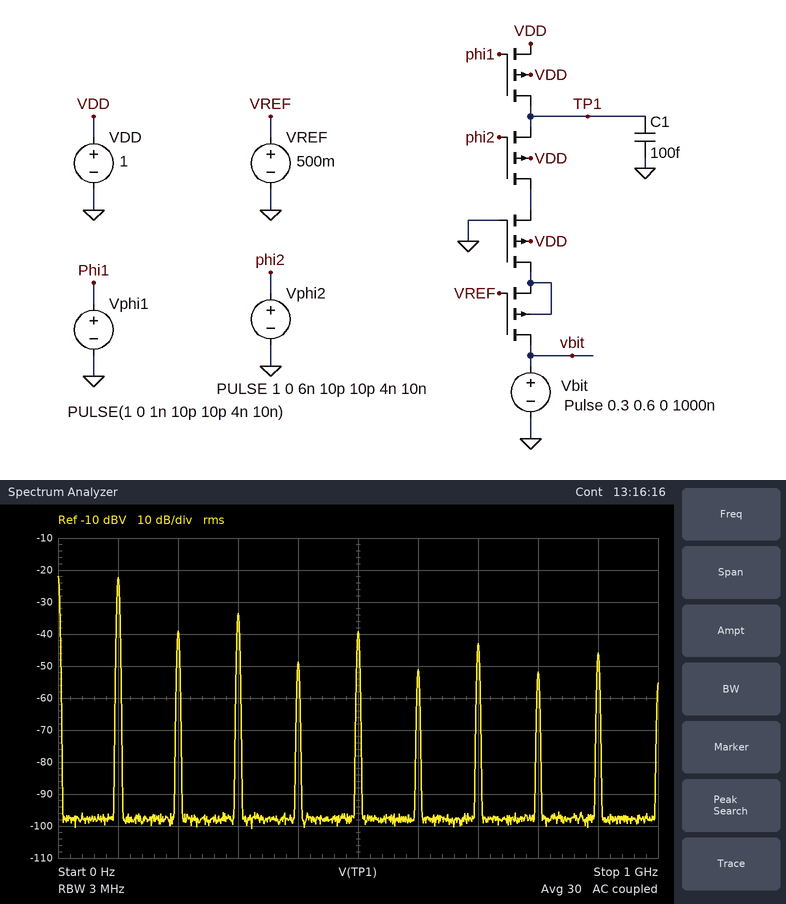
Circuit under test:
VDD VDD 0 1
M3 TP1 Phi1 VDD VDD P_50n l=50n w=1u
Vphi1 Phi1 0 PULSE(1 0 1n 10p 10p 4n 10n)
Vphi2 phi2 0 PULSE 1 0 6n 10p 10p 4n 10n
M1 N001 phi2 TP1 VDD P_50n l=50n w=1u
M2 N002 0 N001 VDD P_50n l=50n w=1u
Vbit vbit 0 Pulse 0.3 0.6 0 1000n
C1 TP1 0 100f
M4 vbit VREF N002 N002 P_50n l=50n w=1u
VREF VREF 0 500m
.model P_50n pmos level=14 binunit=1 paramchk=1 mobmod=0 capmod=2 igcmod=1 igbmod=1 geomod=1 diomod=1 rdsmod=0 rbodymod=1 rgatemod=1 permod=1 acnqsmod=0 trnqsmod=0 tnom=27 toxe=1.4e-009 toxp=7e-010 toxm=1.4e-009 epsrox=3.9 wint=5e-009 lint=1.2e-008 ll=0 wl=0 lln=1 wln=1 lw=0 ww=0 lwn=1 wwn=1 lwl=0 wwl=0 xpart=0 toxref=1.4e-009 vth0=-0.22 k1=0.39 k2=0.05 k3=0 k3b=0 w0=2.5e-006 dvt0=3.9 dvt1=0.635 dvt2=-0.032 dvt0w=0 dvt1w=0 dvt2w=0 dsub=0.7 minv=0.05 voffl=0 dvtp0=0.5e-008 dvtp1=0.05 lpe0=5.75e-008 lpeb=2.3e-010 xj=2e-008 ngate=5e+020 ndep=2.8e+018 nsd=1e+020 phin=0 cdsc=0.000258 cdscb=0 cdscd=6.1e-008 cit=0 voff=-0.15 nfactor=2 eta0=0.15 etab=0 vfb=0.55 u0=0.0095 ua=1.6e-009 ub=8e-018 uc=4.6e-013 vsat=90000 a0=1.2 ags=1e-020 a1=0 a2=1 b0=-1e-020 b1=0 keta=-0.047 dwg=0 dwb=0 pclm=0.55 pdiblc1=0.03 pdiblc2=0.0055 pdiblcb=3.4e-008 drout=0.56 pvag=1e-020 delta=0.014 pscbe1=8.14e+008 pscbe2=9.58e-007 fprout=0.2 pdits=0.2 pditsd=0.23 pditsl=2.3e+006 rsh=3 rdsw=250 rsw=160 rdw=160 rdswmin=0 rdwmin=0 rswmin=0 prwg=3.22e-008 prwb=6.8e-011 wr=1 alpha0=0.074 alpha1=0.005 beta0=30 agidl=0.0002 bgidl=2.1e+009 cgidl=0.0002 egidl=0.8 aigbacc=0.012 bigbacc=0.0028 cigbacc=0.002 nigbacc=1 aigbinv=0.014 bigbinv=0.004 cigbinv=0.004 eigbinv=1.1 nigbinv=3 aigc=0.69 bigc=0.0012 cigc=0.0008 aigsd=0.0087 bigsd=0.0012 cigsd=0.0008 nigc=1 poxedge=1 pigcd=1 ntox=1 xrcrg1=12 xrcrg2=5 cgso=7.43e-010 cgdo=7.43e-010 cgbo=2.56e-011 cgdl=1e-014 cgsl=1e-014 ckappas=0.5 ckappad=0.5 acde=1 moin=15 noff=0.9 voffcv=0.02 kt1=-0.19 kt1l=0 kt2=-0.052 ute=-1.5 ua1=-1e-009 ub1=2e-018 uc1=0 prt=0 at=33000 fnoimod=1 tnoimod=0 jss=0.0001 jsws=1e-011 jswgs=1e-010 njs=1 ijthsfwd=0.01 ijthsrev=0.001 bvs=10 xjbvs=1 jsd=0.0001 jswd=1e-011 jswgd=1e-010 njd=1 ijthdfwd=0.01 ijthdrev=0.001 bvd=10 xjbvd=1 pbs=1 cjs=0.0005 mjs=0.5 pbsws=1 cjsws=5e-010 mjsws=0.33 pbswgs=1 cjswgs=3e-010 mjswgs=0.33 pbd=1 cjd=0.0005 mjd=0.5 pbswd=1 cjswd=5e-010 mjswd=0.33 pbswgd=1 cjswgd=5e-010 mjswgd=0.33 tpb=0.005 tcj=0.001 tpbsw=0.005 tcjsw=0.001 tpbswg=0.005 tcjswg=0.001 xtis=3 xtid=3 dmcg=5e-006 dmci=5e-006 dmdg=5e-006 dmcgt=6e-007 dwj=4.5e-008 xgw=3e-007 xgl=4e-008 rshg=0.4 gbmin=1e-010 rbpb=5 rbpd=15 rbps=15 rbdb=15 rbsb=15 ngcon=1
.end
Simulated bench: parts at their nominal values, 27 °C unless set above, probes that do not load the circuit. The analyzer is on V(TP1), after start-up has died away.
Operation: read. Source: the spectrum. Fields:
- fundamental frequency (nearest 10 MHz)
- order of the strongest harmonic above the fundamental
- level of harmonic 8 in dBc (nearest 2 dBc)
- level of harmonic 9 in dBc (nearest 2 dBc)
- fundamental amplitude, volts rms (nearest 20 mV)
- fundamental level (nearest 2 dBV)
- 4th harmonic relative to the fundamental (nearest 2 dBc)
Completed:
100 MHz
3
-30 dBc
-24 dBc
80 mV
-22 dBV
-26 dBc
